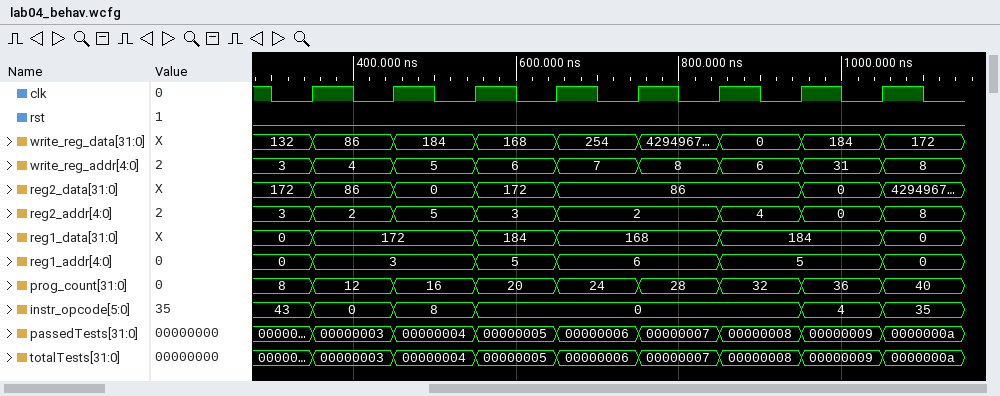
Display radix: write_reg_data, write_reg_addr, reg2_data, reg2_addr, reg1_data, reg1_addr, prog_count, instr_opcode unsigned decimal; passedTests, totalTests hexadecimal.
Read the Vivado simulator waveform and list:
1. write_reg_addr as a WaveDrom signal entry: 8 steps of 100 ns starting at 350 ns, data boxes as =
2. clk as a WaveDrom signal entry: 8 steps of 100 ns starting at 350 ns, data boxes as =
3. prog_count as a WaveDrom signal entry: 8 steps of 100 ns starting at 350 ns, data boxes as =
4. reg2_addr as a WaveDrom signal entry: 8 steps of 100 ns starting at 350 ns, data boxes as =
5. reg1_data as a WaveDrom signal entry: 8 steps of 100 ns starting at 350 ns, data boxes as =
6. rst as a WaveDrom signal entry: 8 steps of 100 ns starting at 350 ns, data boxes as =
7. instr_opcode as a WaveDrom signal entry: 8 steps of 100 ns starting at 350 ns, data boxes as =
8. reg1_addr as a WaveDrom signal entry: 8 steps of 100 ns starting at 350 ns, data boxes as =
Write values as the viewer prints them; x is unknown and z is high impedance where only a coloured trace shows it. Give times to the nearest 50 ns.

{name: 'write_reg_addr', wave: '========', data: '4 5 6 7 8 6 31 8'}
{name: 'clk', wave: 'p.......'}
{name: 'prog_count', wave: '========', data: '12 16 20 24 28 32 36 40'}
{name: 'reg2_addr', wave: '====.===', data: '2 5 3 2 4 0 8'}
{name: 'reg1_data', wave: '=.==.=.=', data: '172 184 168 184 0'}
{name: 'rst', wave: '0.......'}
{name: 'instr_opcode', wave: '===...==', data: '0 8 0 4 35'}
{name: 'reg1_addr', wave: '=.==.=.=', data: '3 5 6 5 0'}
